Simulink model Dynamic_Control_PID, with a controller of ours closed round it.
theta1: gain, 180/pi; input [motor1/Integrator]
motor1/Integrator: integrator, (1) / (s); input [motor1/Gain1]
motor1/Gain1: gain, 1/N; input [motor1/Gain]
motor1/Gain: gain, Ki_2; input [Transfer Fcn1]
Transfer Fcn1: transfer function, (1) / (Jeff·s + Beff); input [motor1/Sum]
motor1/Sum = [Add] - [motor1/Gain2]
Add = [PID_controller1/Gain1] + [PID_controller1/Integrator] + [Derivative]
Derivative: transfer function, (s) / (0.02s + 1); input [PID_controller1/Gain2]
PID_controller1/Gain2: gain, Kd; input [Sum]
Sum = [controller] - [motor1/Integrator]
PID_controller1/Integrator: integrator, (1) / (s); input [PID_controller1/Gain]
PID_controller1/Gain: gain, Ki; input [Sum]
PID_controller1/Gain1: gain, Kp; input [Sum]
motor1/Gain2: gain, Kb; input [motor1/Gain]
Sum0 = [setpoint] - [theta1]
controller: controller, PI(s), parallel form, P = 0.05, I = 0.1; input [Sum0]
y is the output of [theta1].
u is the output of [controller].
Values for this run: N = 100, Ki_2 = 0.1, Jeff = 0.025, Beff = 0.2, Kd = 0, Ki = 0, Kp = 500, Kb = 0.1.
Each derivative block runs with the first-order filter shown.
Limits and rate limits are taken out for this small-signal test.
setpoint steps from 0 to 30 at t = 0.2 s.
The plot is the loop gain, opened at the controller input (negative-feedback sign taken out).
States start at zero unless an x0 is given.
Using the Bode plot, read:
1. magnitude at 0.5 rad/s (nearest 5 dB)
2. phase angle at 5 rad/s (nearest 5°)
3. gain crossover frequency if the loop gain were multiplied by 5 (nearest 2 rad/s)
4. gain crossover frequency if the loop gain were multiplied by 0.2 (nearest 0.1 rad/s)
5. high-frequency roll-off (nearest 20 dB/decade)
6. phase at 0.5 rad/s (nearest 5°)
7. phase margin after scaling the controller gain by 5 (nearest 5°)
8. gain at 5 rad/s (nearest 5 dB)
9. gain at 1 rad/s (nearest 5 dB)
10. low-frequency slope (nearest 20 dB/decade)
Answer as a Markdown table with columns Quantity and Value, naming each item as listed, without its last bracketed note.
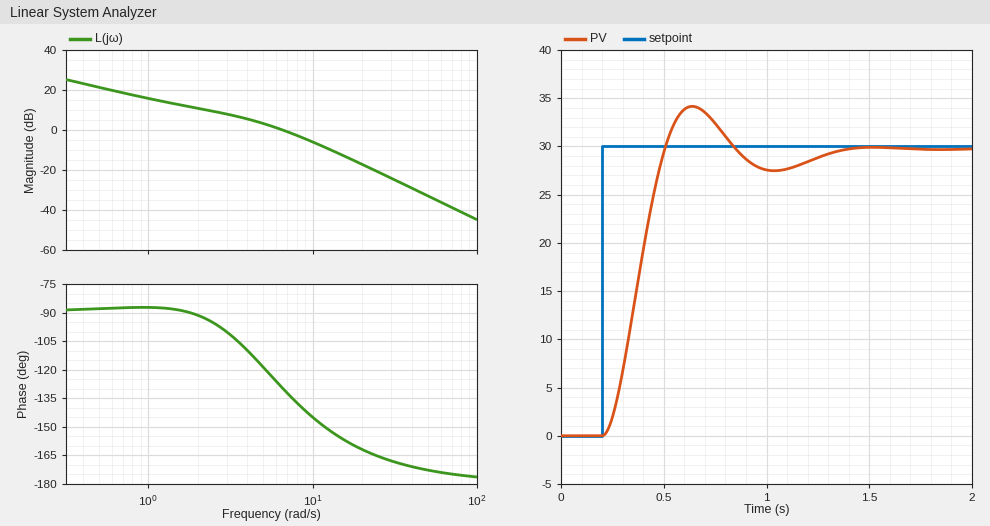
| Quantity | Value |
|---|---|
| magnitude at 0.5 rad/s | 20 dB |
| phase angle at 5 rad/s | -120° |
| gain crossover frequency if the loop gain were multiplied by 5 | 16 rad/s |
| gain crossover frequency if the loop gain were multiplied by 0.2 | 1.3 rad/s |
| high-frequency roll-off | -40 dB/decade |
| phase at 0.5 rad/s | -90° |
| phase margin after scaling the controller gain by 5 | 20° |
| gain at 5 rad/s | 5 dB |
| gain at 1 rad/s | 15 dB |
| low-frequency slope | -20 dB/decade |
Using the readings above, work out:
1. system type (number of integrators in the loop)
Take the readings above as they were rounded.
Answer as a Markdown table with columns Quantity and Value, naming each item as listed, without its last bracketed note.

| Quantity | Value |
|---|---|
| system type | 1 |
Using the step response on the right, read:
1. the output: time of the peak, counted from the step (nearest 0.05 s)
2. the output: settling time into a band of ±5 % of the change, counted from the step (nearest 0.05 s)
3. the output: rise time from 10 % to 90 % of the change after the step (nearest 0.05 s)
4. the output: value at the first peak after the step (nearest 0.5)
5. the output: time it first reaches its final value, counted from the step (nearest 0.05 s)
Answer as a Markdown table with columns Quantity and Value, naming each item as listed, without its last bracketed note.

| Quantity | Value |
|---|---|
| the output: time of the peak, counted from the step | 0.45 s |
| the output: settling time into a band of ±5 % of the change, counted from the step | 1.00 s |
| the output: rise time from 10 % to 90 % of the change after the step | 0.20 s |
| the output: value at the first peak after the step | 34.0 |
| the output: time it first reaches its final value, counted from the step | 0.30 s |
